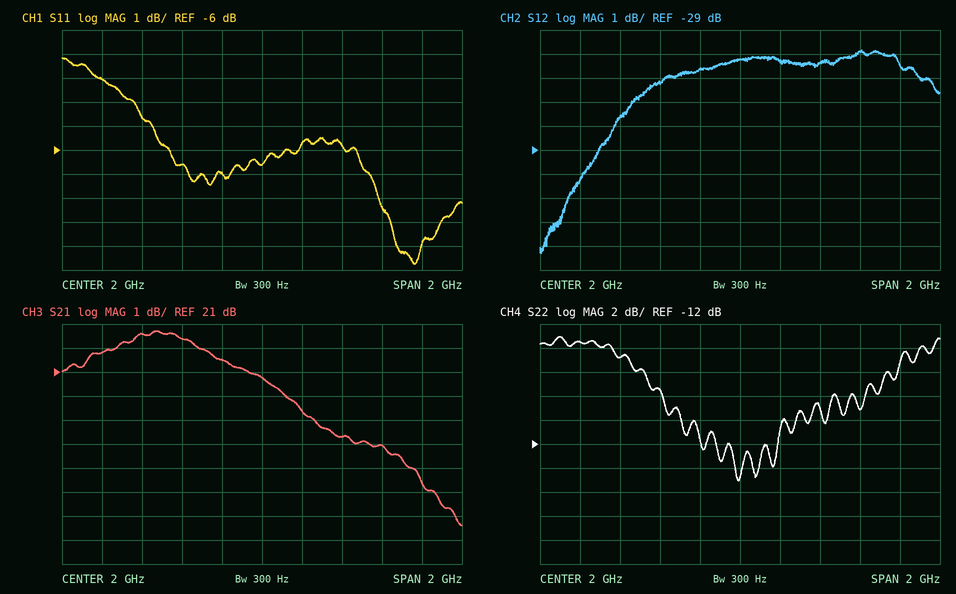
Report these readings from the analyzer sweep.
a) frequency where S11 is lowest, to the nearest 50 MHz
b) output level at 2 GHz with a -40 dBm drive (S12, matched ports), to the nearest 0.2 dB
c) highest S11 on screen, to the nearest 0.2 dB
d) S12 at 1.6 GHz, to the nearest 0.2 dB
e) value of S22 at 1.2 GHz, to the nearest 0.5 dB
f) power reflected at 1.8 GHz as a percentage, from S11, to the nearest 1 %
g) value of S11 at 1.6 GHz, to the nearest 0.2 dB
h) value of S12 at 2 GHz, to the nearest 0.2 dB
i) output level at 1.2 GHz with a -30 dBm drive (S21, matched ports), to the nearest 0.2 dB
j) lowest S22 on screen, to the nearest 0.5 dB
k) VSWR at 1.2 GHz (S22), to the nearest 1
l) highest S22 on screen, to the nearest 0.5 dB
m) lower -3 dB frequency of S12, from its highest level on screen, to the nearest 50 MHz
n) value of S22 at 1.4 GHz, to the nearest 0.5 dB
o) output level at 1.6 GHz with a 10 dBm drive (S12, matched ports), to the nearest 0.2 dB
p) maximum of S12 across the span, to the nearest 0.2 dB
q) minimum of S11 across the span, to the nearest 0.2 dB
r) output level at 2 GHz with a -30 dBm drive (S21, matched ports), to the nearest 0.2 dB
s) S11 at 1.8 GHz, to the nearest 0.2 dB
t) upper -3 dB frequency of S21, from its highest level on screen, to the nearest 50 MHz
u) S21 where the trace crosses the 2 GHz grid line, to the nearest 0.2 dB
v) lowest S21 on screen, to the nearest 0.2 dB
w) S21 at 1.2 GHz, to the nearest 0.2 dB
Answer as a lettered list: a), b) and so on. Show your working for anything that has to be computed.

a) 2.75 GHz
b) -40 dBm + (-25.2 dB) = -65.2 dBm
c) -2.2 dB
d) -26.2 dB
e) -3.5 dB
f) 10^(-7/10) ≈ 20 %
g) -6.6 dB
h) -25.2 dB
i) -30 dBm + (21.8 dB) = -8.2 dBm
j) -15.0 dB
k) |Γ| = 10^(-3.5/20) = 0.6683; VSWR = (1 + 0.6683)/(1 − 0.6683) ≈ 5
l) -3.0 dB
m) 1.40 GHz
n) -5.0 dB
o) 10 dBm + (-26.2 dB) = -16.2 dBm
p) -24.8 dB
q) -10.8 dB
r) -30 dBm + (20.8 dB) = -9.2 dBm
s) -7.0 dB
t) 2.15 GHz
u) 20.8 dB
v) 14.6 dB
w) 21.8 dB
